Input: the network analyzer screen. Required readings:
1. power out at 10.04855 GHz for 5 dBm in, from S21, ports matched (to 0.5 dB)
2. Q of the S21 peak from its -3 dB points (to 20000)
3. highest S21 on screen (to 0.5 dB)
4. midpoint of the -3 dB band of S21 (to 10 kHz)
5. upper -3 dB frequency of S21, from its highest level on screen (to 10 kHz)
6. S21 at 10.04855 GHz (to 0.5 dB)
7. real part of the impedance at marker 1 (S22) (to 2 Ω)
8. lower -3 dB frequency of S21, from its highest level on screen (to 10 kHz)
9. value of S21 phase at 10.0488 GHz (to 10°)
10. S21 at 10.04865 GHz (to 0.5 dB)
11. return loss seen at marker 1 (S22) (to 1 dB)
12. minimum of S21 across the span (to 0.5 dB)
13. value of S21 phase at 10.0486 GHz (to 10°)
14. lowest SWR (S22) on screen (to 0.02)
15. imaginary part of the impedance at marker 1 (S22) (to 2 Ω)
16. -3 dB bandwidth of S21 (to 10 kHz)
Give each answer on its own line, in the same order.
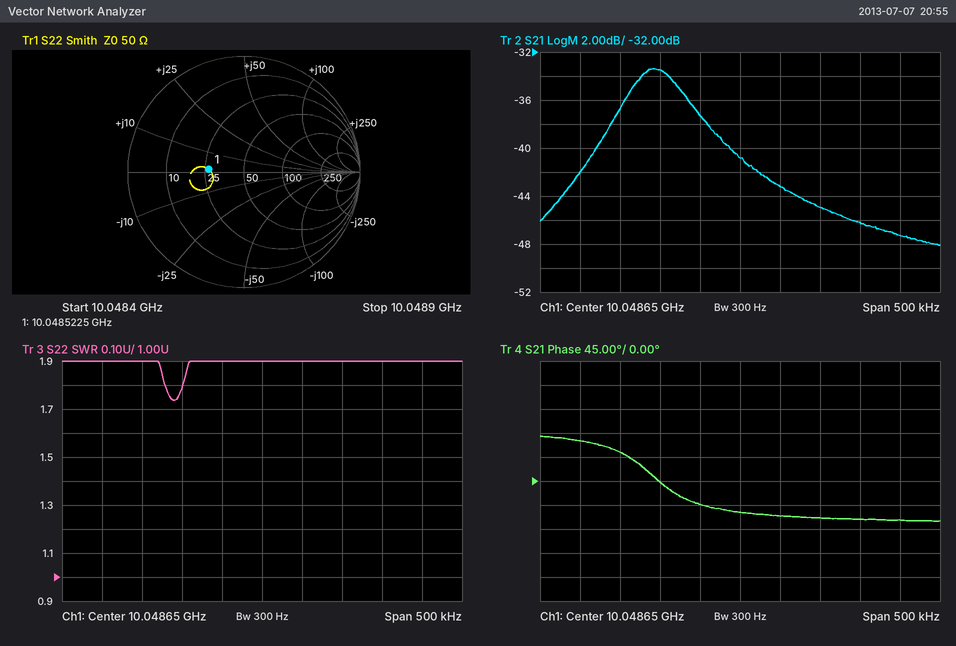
-28.5 dBm
120000
-33.5 dB
10.04855 GHz
10.04859 GHz
-33.5 dB
26 Ω
10.04850 GHz
-70°
-41.0 dB
10 dB
-48.0 dB
-40°
1.74
+2 Ω
90 kHz
